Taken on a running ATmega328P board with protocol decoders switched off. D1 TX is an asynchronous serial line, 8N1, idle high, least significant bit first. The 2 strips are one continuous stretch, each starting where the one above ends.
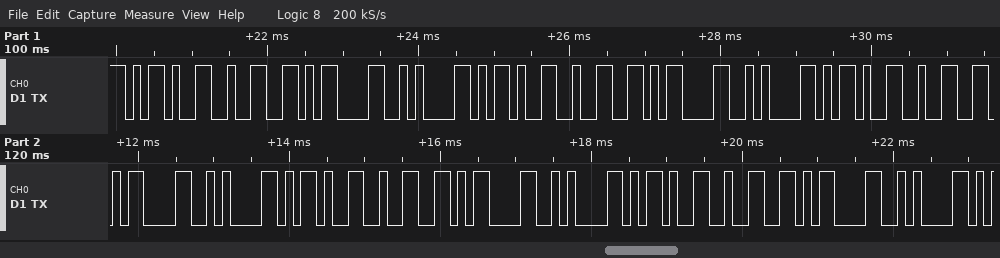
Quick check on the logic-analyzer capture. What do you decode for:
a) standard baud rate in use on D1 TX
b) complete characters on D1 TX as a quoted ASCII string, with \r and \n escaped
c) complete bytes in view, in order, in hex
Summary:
9600 baud
"-2\r\n-2\r\n-2\r\n-2\r\n-2\r\n"
2D 32 0D 0A 2D 32 0D 0A 2D 32 0D 0A 2D 32 0D 0A 2D 32 0D 0A
